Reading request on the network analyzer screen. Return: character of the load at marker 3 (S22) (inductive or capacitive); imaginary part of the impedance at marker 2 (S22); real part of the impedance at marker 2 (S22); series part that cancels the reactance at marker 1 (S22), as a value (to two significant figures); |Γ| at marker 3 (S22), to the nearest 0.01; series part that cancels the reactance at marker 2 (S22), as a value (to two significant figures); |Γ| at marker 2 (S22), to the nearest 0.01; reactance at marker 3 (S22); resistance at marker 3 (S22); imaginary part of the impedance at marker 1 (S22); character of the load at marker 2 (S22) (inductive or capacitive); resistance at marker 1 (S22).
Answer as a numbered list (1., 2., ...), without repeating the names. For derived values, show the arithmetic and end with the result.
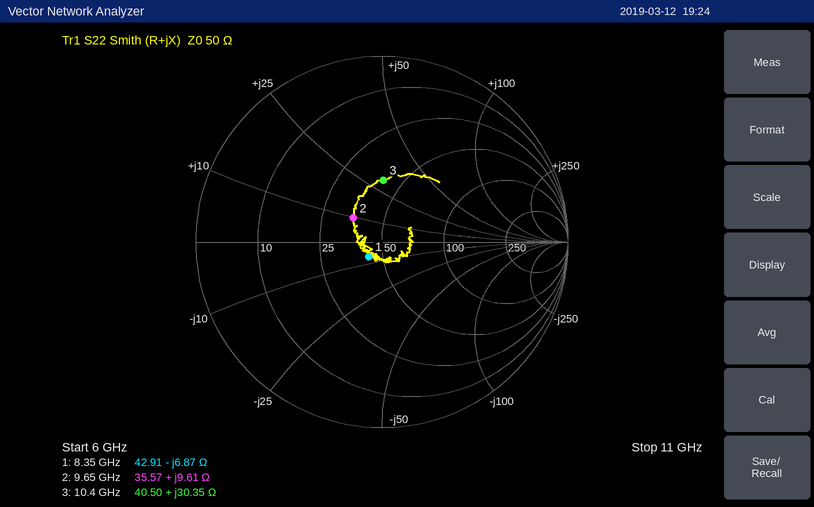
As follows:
1. inductive
2. +9.61 Ω
3. 35.57 Ω
4. L = 6.87 Ω/(2π × 8.35 GHz) ≈ 131 pH, so 130 pH to two significant figures
5. 0.33
6. C = 1/(2π × 9.65 GHz × 9.61 Ω) ≈ 1.7 pF
7. 0.20
8. +30.35 Ω
9. 40.50 Ω
10. -6.87 Ω
11. inductive
12. 42.91 Ω
